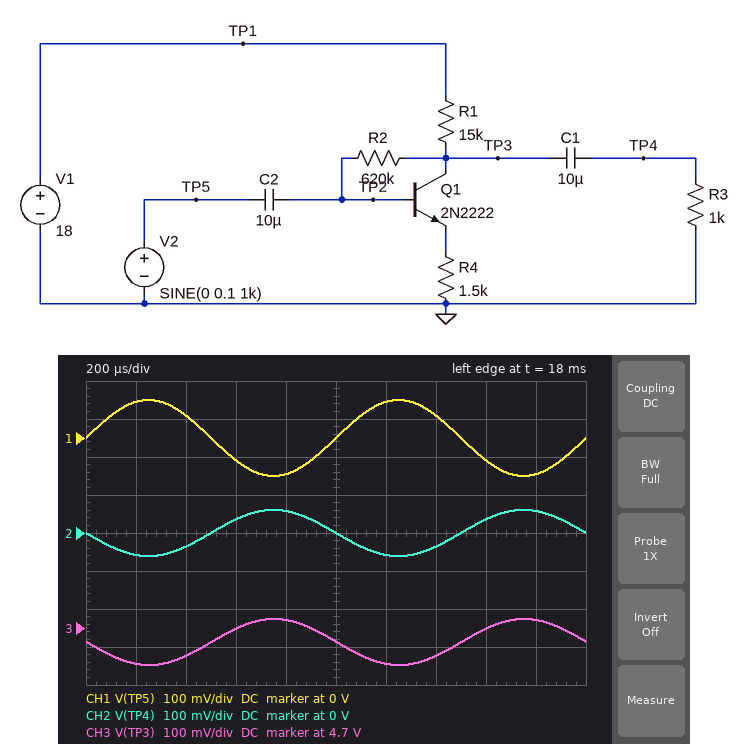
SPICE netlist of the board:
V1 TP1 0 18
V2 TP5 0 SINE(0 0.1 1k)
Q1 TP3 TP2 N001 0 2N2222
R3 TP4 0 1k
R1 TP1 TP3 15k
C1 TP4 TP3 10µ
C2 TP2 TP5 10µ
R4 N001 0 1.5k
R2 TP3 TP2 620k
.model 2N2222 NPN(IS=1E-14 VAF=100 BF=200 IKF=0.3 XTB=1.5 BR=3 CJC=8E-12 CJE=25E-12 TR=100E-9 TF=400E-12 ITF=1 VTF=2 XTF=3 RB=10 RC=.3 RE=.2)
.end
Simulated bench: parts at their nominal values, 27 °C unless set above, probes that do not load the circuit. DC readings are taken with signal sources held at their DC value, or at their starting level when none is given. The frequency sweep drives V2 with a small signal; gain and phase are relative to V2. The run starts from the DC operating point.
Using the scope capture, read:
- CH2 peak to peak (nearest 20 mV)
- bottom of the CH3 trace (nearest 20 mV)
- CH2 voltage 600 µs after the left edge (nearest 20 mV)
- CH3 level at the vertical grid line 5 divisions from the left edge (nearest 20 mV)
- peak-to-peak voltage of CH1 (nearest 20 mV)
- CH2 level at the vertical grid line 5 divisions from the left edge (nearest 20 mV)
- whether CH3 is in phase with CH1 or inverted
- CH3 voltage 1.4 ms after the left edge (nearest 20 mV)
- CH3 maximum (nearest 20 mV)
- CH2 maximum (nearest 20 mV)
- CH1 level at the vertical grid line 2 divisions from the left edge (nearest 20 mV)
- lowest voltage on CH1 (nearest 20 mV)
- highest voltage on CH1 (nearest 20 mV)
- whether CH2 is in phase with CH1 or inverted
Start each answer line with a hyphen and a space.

- 120 mV
- 4.60 V
- 40 mV
- 4.66 V
- 200 mV
- 0 V
- inverted
- 4.62 V
- 4.72 V
- 60 mV
- 60 mV
- -100 mV
- 100 mV
- inverted
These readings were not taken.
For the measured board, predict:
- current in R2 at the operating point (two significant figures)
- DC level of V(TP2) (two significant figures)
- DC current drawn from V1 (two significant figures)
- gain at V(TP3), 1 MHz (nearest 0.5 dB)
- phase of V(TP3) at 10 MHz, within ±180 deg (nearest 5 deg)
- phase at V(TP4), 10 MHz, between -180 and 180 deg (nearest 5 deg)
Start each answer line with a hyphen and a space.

- 4.3 µA
- 2.0 V
- 890 µA
- -4.5 dB
- 135 deg
- 135 deg
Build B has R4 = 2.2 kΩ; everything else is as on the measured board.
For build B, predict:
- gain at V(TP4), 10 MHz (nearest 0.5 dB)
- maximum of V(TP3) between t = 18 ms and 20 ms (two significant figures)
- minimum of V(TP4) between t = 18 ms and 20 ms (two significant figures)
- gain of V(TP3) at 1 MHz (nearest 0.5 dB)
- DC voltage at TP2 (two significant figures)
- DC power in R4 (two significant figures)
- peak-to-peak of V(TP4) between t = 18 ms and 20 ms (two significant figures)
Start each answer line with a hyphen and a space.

- -6.0 dB
- 5.2 V
- -42 mV
- -7.5 dB
- 2.5 V
- 1.6 mW
- 83 mV
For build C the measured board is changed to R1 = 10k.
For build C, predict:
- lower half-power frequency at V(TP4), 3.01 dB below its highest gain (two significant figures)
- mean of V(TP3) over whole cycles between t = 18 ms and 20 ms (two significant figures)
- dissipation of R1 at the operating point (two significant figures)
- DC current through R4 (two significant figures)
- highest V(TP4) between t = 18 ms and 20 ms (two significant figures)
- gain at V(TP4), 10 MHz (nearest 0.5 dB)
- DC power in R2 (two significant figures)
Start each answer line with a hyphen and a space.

- 19 MHz
- 6.0 V
- 14 mW
- 1.2 mA
- 59 mV
- -4.0 dB
- 21 µW
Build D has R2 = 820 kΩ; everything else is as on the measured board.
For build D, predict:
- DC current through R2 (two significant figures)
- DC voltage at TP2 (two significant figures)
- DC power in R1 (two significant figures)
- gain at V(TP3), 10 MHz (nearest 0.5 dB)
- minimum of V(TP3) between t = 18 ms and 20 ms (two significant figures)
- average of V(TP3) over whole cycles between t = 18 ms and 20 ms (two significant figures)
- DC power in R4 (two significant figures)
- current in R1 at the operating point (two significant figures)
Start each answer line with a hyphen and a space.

- 4.1 µA
- 1.9 V
- 11 mW
- -3.5 dB
- 5.2 V
- 5.3 V
- 1.1 mW
- 850 µA
